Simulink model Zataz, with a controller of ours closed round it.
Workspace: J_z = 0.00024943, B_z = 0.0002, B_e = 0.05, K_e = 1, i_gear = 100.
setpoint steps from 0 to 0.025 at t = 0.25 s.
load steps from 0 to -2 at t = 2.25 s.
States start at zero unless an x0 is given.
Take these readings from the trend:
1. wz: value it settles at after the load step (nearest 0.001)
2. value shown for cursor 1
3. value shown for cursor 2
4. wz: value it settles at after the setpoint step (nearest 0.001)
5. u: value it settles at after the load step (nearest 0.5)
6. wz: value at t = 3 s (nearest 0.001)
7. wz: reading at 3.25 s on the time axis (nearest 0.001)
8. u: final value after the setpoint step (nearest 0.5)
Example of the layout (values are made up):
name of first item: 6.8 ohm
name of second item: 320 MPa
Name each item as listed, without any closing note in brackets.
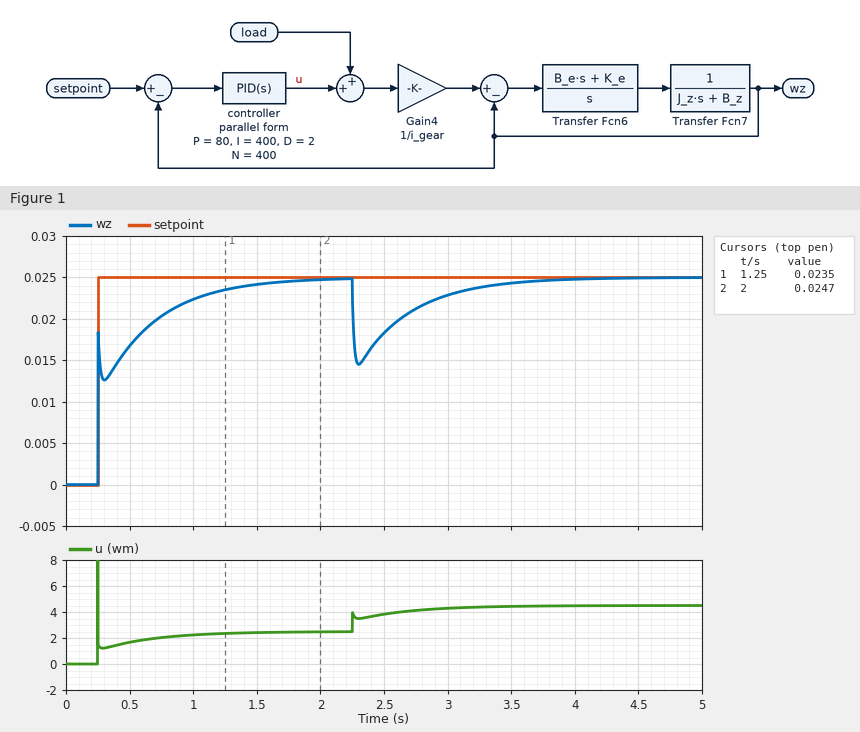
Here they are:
wz: value it settles at after the load step: 0.025
value shown for cursor 1: 0.0235
value shown for cursor 2: 0.0247
wz: value it settles at after the setpoint step: 0.025
u: value it settles at after the load step: 4.5
wz: value at t = 3 s: 0.023
wz: reading at 3.25 s on the time axis: 0.024
u: final value after the setpoint step: 2.5
